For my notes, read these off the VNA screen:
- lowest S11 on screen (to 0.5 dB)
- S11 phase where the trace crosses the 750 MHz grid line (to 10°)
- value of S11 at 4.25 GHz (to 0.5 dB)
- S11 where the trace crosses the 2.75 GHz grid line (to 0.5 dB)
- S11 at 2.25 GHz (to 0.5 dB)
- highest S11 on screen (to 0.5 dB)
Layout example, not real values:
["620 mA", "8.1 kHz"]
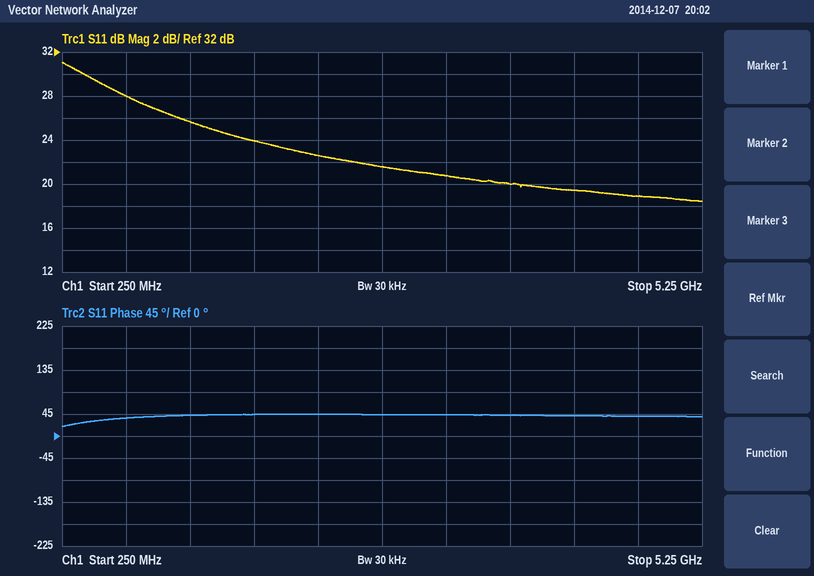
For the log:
["18.5 dB", "40°", "19.5 dB", "21.5 dB", "22.5 dB", "31.0 dB"]
